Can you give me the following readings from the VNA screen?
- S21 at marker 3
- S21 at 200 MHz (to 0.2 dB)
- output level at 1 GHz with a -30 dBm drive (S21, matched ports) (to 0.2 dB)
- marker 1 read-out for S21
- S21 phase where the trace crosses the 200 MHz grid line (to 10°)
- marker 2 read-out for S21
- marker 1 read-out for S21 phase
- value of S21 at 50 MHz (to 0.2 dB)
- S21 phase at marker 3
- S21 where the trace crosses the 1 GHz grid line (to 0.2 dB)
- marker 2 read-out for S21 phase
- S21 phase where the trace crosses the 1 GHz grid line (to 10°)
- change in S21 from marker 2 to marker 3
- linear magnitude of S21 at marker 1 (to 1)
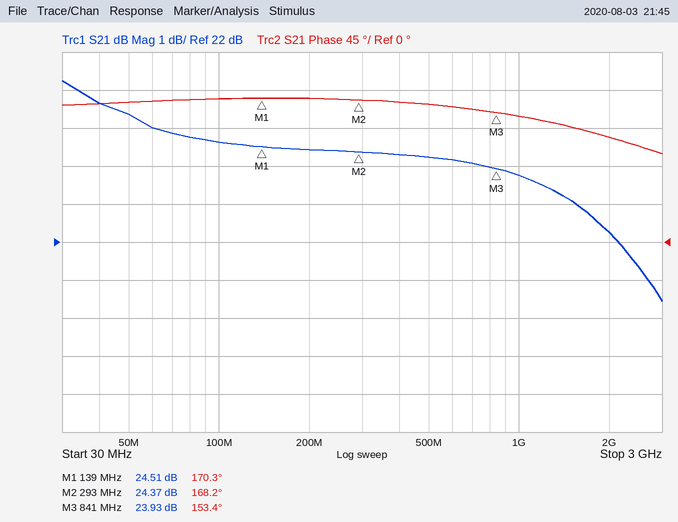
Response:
23.93 dB
24.4 dB
-6.2 dBm
24.51 dB
170°
24.37 dB
170.3°
25.4 dB
153.4°
23.8 dB
168.2°
150°
-0.44 dB
17
